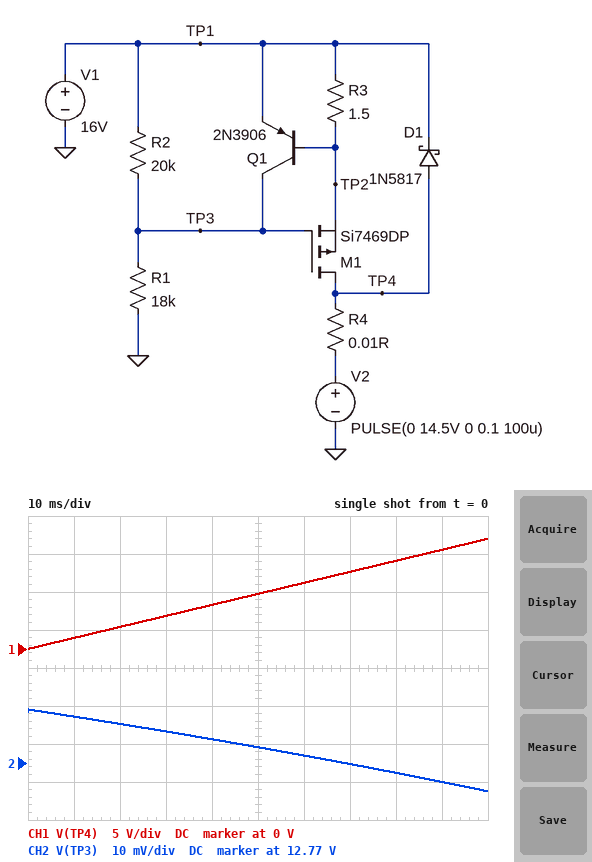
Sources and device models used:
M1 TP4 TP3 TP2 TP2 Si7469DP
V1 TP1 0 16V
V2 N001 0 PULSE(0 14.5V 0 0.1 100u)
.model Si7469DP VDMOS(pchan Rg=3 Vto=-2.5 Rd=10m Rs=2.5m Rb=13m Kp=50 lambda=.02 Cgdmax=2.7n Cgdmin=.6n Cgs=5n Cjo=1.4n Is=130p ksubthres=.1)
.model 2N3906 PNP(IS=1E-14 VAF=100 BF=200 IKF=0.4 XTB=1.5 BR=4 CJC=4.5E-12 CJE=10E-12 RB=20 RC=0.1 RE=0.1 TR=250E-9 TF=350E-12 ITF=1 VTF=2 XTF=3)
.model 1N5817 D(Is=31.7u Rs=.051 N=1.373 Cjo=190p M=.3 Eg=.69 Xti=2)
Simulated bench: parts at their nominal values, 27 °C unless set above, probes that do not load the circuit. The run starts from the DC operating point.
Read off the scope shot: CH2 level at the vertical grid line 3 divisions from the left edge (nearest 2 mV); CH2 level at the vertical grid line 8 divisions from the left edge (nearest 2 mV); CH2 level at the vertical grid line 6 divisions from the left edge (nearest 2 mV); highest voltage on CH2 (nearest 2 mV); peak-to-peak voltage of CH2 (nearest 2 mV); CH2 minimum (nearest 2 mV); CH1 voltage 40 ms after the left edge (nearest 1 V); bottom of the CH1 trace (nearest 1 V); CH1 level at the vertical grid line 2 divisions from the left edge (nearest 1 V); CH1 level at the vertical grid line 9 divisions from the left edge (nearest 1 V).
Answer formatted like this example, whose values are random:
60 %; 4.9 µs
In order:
12.778 V; 12.768 V; 12.772 V; 12.784 V; 22 mV; 12.762 V; 6 V; 0 V; 3 V; 13 V
